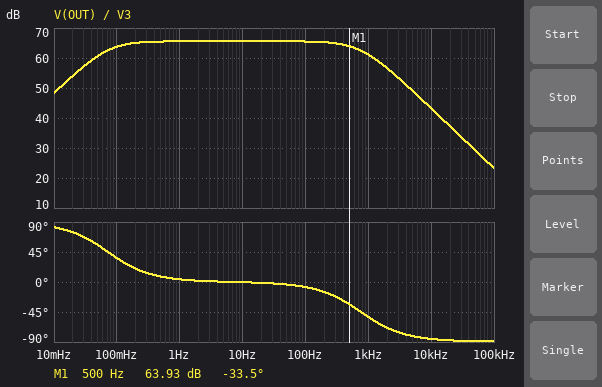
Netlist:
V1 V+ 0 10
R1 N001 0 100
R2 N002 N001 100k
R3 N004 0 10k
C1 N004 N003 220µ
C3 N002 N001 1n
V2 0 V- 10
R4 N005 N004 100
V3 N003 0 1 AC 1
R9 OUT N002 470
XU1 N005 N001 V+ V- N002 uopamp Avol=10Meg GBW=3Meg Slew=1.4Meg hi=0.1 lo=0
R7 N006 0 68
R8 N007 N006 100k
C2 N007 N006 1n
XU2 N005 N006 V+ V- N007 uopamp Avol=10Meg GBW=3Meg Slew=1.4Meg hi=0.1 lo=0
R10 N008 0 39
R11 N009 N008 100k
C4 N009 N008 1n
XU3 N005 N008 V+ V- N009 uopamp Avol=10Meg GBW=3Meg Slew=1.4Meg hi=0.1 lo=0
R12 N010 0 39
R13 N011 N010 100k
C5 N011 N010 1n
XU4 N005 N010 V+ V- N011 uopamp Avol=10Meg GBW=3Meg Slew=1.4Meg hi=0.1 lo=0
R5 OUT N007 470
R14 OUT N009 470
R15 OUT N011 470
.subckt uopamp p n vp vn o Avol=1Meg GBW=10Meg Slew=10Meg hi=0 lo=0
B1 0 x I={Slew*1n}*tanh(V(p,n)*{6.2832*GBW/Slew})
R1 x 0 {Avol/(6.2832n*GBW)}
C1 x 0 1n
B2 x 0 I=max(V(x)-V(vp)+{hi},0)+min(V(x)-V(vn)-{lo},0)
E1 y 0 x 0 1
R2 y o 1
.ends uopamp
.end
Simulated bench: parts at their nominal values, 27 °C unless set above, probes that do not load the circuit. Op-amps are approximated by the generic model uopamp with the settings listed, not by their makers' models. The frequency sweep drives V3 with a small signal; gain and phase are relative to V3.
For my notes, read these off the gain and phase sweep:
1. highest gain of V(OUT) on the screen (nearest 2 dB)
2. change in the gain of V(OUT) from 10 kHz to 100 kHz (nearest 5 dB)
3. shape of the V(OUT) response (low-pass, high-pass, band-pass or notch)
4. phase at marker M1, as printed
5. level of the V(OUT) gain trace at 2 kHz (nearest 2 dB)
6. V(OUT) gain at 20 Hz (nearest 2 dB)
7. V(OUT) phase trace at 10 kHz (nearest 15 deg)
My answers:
66 dB
-20 dB
band-pass
-33.5 deg
56 dB
66 dB
-90 deg
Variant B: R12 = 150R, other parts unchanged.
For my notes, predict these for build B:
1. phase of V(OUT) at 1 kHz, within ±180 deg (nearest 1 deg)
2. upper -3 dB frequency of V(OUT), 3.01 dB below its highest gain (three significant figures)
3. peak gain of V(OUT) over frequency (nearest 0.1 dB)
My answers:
-49 deg
816 Hz
63.1 dB
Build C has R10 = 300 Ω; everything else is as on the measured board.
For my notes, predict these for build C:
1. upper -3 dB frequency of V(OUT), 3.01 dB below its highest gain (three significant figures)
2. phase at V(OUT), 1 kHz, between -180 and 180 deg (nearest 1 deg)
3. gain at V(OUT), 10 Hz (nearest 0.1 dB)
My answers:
804 Hz
-50 deg
62.6 dB
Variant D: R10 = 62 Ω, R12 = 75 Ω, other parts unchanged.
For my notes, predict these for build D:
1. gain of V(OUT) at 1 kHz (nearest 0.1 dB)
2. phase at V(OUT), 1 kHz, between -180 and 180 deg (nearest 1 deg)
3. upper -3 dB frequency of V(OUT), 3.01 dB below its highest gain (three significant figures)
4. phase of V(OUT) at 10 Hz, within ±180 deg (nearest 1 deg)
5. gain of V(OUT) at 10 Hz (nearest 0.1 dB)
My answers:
59.2 dB
-47 deg
915 Hz
0 deg
62.6 dB
